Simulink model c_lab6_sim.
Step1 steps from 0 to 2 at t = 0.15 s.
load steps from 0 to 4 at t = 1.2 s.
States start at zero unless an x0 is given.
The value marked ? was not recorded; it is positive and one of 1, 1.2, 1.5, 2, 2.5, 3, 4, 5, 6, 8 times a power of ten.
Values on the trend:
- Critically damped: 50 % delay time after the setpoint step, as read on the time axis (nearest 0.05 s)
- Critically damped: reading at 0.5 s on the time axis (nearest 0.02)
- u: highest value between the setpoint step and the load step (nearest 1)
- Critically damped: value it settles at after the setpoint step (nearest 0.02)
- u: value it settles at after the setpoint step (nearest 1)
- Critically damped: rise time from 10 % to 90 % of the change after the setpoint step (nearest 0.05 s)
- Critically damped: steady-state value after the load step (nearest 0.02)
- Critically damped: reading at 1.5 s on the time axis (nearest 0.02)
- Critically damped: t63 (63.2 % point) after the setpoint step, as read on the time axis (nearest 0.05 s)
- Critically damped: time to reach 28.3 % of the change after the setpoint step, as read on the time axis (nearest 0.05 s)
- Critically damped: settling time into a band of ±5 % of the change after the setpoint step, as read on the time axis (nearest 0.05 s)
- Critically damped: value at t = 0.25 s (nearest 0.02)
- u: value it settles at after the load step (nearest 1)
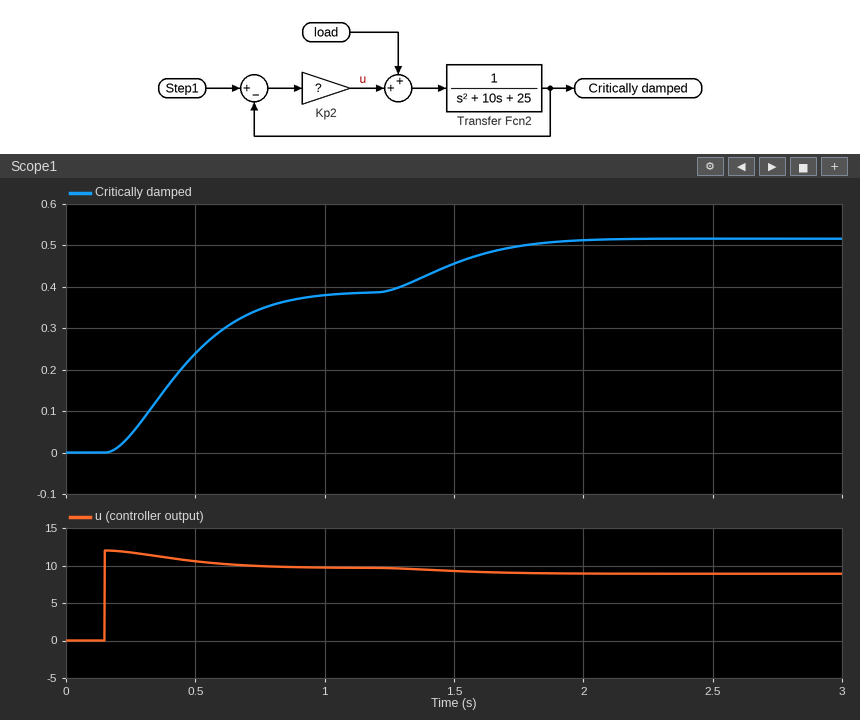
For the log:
0.45 s
0.24
12
0.38
10
0.50 s
0.52
0.46
0.50 s
0.35 s
0.85 s
0.04
9
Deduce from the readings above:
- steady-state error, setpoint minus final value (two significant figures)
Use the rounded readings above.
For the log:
1.6
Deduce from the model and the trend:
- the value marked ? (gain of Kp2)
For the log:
6
